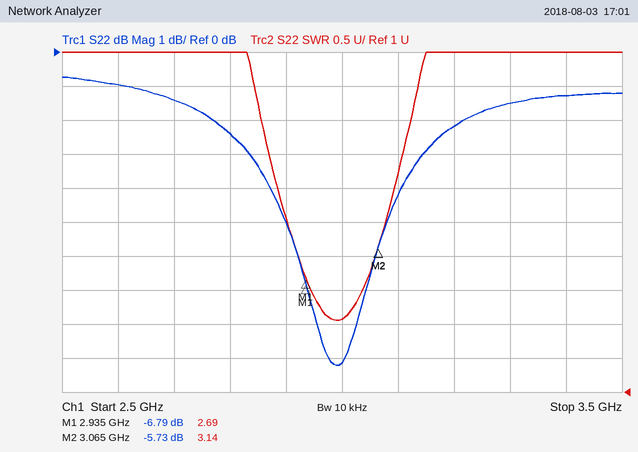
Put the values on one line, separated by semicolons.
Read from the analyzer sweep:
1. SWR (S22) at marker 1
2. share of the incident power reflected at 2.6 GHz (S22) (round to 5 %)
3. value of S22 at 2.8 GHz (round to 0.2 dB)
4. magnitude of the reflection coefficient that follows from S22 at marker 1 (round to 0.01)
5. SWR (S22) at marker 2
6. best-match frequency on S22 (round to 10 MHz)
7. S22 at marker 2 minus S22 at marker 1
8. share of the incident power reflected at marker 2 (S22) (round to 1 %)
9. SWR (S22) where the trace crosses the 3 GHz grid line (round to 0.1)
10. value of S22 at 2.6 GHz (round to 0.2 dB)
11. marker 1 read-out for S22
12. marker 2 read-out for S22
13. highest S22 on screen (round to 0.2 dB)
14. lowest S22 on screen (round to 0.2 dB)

2.69; 80 %; -2.4 dB; 0.46; 3.14; 2.99 GHz; 1.06 dB; 27 %; 2.1; -1.0 dB; -6.79 dB; -5.73 dB; -0.8 dB; -9.2 dB
